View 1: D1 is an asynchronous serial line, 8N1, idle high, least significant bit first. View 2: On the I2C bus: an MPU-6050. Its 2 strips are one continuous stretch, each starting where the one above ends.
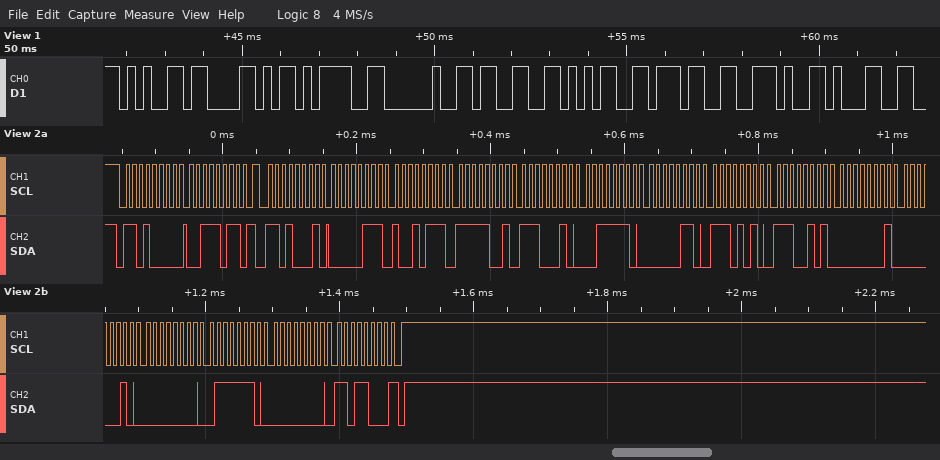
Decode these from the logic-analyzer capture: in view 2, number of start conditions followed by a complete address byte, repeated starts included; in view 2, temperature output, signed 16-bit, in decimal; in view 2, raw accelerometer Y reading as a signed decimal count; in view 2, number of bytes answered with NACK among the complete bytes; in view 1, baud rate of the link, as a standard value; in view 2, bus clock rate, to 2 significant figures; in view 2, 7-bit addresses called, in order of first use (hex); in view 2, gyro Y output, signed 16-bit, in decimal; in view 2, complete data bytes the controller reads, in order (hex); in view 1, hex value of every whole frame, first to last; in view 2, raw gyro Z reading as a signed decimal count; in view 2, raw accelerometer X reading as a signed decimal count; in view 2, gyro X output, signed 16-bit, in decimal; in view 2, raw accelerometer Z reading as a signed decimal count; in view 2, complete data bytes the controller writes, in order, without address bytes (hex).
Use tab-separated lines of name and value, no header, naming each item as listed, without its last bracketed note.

in view 2, number of start conditions followed by a complete address byte, repeated starts included	2
in view 2, temperature output, signed 16-bit, in decimal	-5403
in view 2, raw accelerometer Y reading as a signed decimal count	-1566
in view 2, number of bytes answered with NACK among the complete bytes	1
in view 1, baud rate of the link, as a standard value	4800 baud
in view 2, bus clock rate, to 2 significant figures	100 kHz
in view 2, 7-bit addresses called, in order of first use	0x68
in view 2, gyro Y output, signed 16-bit, in decimal	126
in view 2, complete data bytes the controller reads, in order	07 97 F9 E2 3E 06 EA E5 01 02 00 7E 00 D8
in view 1, hex value of every whole frame, first to last	65 58 3D 20 33 35 37 2E 31
in view 2, raw gyro Z reading as a signed decimal count	216
in view 2, raw accelerometer X reading as a signed decimal count	1943
in view 2, gyro X output, signed 16-bit, in decimal	258
in view 2, raw accelerometer Z reading as a signed decimal count	15878
in view 2, complete data bytes the controller writes, in order, without address bytes	3B
